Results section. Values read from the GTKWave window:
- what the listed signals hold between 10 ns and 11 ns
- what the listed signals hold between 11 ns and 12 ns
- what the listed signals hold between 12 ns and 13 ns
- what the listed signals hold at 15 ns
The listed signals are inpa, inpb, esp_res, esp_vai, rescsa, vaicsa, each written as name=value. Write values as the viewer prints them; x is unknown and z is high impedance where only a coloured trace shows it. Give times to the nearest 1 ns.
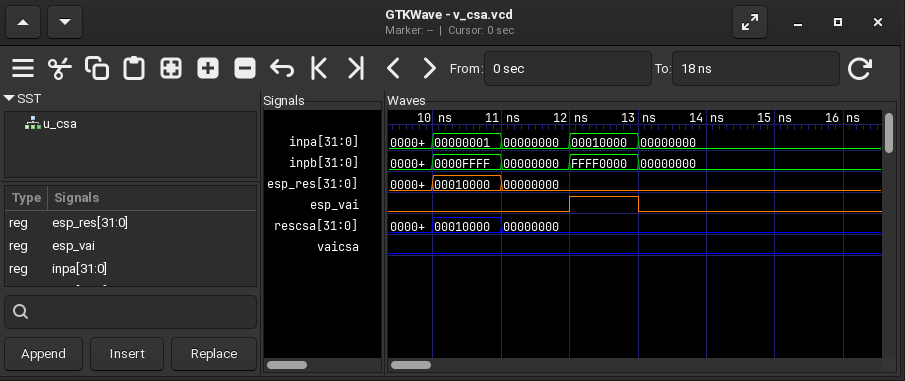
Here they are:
inpa=00000001, inpb=0000FFFF, esp_res=00010000, esp_vai=0, rescsa=00010000, vaicsa=0
inpa=00000000, inpb=00000000, esp_res=00000000, esp_vai=0, rescsa=00000000, vaicsa=0
inpa=00010000, inpb=FFFF0000, esp_res=00000000, esp_vai=1, rescsa=00000000, vaicsa=0
inpa=00000000, inpb=00000000, esp_res=00000000, esp_vai=0, rescsa=00000000, vaicsa=0
